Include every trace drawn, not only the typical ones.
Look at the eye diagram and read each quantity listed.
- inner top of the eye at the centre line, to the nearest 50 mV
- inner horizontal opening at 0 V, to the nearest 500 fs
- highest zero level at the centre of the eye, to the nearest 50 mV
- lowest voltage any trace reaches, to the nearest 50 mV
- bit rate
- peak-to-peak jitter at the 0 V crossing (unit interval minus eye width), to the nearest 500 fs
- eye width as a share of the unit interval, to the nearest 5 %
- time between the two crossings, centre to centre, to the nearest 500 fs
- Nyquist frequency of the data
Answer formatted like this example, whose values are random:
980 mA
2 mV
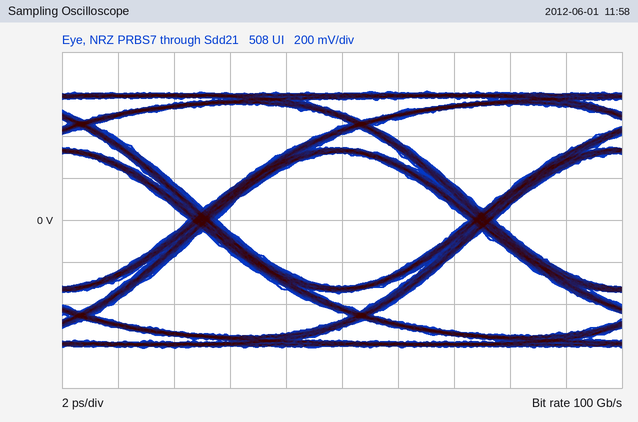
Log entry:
300 mV
9.0 ps
-300 mV
-600 mV
100 Gb/s
1.0 ps
90 %
10.0 ps
50 GHz
